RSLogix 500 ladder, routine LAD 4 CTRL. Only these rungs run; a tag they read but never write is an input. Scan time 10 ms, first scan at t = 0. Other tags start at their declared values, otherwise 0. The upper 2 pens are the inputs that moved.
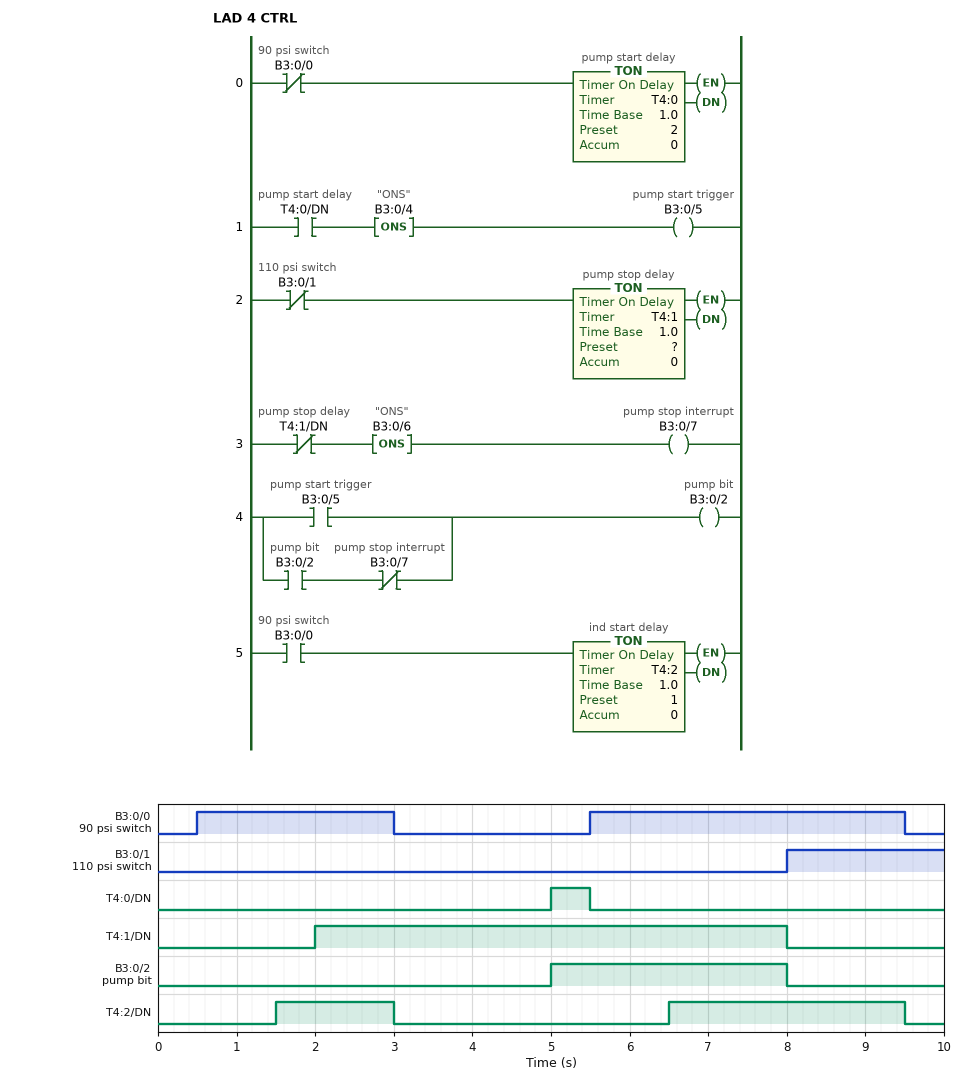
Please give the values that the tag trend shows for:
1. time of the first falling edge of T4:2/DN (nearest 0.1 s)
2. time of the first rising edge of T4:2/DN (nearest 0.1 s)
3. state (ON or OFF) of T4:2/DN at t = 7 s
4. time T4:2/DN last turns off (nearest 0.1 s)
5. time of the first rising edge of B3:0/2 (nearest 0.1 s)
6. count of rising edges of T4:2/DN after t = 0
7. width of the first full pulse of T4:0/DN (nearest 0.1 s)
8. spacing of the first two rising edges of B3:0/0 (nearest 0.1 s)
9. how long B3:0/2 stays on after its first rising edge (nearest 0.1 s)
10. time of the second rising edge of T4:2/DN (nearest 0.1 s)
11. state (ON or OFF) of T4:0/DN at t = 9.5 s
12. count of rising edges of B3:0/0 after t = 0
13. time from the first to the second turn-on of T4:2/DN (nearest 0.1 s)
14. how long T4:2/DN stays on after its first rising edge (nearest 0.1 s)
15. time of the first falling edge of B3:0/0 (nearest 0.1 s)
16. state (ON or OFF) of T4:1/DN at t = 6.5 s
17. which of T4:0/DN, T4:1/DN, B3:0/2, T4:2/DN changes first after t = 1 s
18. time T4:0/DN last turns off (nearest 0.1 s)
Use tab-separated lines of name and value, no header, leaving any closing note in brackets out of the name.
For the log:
time of the first falling edge of T4:2/DN	3.0 s
time of the first rising edge of T4:2/DN	1.5 s
state (ON or OFF) of T4:2/DN at t = 7 s	ON
time T4:2/DN last turns off	9.5 s
time of the first rising edge of B3:0/2	5.0 s
count of rising edges of T4:2/DN after t = 0	2
width of the first full pulse of T4:0/DN	0.5 s
spacing of the first two rising edges of B3:0/0	5.0 s
how long B3:0/2 stays on after its first rising edge	3.0 s
time of the second rising edge of T4:2/DN	6.5 s
state (ON or OFF) of T4:0/DN at t = 9.5 s	OFF
count of rising edges of B3:0/0 after t = 0	2
time from the first to the second turn-on of T4:2/DN	5.0 s
how long T4:2/DN stays on after its first rising edge	1.5 s
time of the first falling edge of B3:0/0	3.0 s
state (ON or OFF) of T4:1/DN at t = 6.5 s	ON
which of T4:0/DN, T4:1/DN, B3:0/2, T4:2/DN changes first after t = 1 s	T4:2/DN
time T4:0/DN last turns off	5.5 s
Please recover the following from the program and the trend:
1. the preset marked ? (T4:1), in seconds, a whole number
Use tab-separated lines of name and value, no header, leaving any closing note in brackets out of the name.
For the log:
the preset marked ? (T4:1), in seconds, a whole number	2 s
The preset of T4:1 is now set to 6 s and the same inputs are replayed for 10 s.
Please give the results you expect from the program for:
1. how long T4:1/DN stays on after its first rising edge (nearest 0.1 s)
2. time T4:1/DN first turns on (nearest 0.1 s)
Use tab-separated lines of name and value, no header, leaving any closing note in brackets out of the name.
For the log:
how long T4:1/DN stays on after its first rising edge	2.0 s
time T4:1/DN first turns on	6.0 s
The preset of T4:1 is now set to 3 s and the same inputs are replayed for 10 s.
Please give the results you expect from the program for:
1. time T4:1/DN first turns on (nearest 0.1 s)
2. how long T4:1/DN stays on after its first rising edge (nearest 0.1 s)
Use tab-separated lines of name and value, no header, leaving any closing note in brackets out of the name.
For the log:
time T4:1/DN first turns on	3.0 s
how long T4:1/DN stays on after its first rising edge	5.0 s
